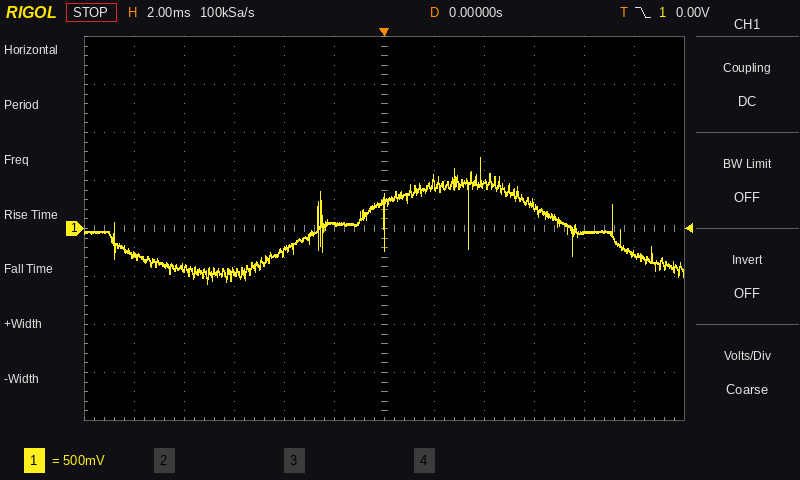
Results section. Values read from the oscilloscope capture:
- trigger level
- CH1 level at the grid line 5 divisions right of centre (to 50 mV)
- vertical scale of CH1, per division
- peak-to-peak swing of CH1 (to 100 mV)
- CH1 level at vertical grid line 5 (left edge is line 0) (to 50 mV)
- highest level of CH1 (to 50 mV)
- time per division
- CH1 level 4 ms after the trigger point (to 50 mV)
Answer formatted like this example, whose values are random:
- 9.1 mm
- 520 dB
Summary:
- 0.00 V
- -250 mV
- 500 mV
- 1.30 V
- 50 mV
- 750 mV
- 2 ms
- 450 mV
